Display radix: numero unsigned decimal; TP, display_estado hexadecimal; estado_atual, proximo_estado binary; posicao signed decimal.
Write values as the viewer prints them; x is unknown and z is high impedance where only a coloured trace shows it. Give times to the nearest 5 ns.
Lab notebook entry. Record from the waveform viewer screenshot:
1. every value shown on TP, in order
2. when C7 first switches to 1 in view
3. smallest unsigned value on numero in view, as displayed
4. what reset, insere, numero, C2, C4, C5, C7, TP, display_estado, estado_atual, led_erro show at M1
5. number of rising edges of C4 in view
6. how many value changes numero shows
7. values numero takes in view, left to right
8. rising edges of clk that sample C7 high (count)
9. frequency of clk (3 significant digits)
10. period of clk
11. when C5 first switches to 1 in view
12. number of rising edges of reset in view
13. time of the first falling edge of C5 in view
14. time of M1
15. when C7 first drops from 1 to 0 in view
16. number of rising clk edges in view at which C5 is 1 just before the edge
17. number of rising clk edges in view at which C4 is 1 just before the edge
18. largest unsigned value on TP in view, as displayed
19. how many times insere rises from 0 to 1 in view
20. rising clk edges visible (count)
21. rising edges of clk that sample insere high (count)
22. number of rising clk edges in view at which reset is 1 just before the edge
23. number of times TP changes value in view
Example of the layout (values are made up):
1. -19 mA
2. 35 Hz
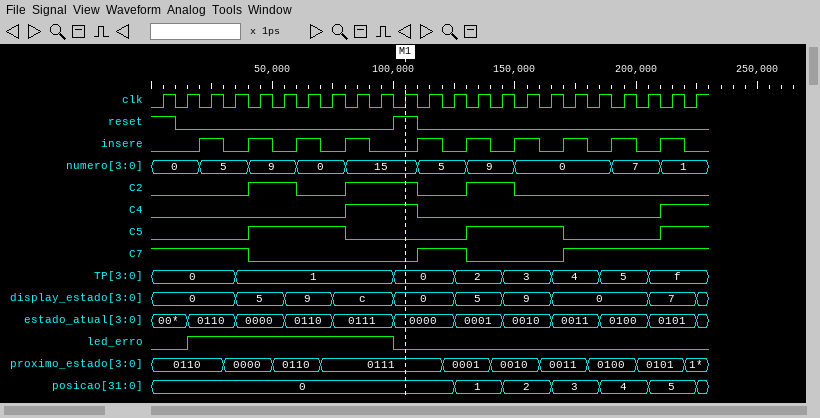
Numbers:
1. 0, 1, 0, 2, 3, 4, 5, f
2. 110 ns
3. 0
4. reset=1, insere=0, numero=15, C2=1, C4=1, C5=0, C7=0, TP=0, display_estado=0, estado_atual=0000, led_erro=0
5. 2
6. 9
7. 0, 5, 9, 0, 15, 5, 9, 0, 7, 1
8. 12
9. 100 MHz
10. 10 ns
11. 40 ns
12. 1
13. 80 ns
14. 105 ns
15. 40 ns
16. 10
17. 5
18. f
19. 10
20. 23
21. 10
22. 2
23. 7
